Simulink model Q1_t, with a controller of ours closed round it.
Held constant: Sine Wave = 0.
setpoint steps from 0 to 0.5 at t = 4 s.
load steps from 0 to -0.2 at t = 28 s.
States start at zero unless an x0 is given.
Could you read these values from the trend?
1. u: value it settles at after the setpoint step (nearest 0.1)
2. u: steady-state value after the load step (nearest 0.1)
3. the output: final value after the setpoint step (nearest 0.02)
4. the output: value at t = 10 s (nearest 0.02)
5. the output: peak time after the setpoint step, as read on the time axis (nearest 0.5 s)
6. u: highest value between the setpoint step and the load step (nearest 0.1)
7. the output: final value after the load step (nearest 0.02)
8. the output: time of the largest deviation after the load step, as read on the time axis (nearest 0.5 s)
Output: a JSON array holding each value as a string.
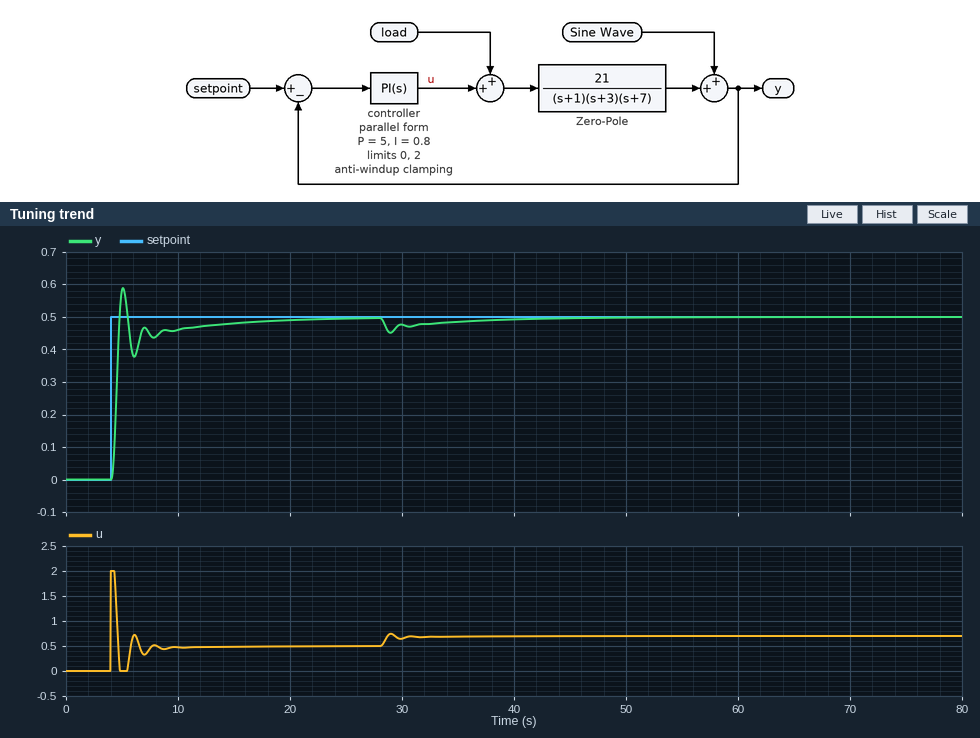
["0.5", "0.7", "0.50", "0.46", "5.0 s", "2.0", "0.50", "29.0 s"]
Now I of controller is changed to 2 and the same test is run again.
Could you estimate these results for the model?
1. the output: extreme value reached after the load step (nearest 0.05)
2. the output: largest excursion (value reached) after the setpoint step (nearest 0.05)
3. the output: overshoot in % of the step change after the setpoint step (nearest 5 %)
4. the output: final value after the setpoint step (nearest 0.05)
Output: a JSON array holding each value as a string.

["0.45", "0.60", "20 %", "0.50"]
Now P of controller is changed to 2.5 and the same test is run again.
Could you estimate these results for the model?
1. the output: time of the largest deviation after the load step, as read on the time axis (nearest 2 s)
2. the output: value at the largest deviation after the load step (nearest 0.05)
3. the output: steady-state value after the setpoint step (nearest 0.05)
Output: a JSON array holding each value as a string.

["30 s", "0.45", "0.50"]
